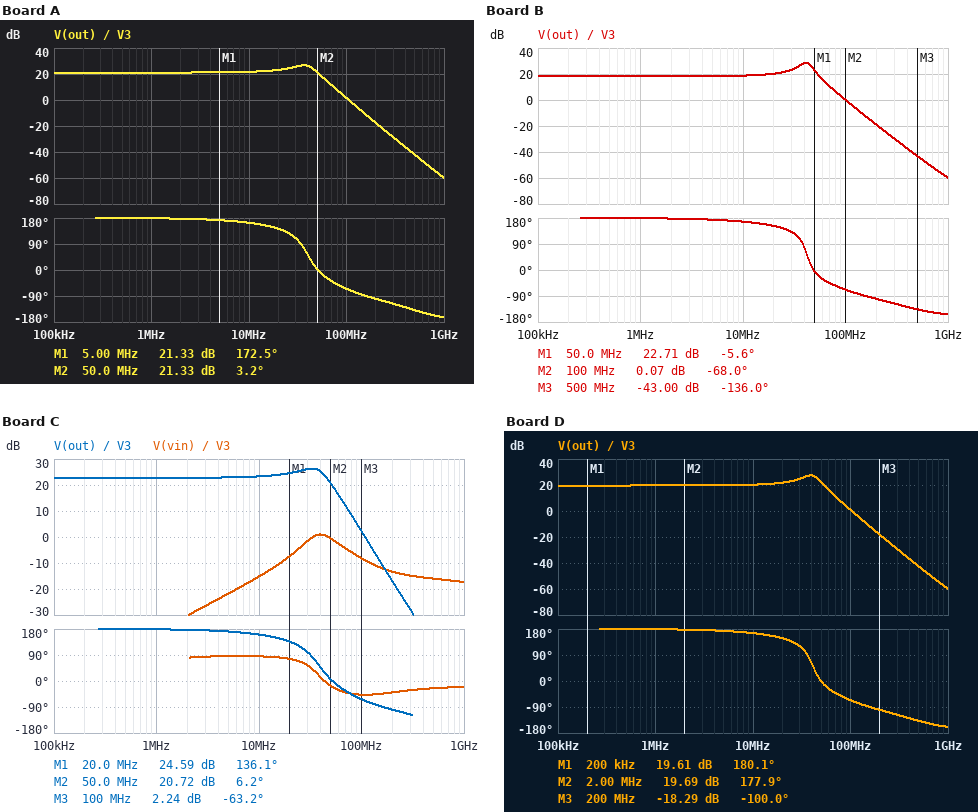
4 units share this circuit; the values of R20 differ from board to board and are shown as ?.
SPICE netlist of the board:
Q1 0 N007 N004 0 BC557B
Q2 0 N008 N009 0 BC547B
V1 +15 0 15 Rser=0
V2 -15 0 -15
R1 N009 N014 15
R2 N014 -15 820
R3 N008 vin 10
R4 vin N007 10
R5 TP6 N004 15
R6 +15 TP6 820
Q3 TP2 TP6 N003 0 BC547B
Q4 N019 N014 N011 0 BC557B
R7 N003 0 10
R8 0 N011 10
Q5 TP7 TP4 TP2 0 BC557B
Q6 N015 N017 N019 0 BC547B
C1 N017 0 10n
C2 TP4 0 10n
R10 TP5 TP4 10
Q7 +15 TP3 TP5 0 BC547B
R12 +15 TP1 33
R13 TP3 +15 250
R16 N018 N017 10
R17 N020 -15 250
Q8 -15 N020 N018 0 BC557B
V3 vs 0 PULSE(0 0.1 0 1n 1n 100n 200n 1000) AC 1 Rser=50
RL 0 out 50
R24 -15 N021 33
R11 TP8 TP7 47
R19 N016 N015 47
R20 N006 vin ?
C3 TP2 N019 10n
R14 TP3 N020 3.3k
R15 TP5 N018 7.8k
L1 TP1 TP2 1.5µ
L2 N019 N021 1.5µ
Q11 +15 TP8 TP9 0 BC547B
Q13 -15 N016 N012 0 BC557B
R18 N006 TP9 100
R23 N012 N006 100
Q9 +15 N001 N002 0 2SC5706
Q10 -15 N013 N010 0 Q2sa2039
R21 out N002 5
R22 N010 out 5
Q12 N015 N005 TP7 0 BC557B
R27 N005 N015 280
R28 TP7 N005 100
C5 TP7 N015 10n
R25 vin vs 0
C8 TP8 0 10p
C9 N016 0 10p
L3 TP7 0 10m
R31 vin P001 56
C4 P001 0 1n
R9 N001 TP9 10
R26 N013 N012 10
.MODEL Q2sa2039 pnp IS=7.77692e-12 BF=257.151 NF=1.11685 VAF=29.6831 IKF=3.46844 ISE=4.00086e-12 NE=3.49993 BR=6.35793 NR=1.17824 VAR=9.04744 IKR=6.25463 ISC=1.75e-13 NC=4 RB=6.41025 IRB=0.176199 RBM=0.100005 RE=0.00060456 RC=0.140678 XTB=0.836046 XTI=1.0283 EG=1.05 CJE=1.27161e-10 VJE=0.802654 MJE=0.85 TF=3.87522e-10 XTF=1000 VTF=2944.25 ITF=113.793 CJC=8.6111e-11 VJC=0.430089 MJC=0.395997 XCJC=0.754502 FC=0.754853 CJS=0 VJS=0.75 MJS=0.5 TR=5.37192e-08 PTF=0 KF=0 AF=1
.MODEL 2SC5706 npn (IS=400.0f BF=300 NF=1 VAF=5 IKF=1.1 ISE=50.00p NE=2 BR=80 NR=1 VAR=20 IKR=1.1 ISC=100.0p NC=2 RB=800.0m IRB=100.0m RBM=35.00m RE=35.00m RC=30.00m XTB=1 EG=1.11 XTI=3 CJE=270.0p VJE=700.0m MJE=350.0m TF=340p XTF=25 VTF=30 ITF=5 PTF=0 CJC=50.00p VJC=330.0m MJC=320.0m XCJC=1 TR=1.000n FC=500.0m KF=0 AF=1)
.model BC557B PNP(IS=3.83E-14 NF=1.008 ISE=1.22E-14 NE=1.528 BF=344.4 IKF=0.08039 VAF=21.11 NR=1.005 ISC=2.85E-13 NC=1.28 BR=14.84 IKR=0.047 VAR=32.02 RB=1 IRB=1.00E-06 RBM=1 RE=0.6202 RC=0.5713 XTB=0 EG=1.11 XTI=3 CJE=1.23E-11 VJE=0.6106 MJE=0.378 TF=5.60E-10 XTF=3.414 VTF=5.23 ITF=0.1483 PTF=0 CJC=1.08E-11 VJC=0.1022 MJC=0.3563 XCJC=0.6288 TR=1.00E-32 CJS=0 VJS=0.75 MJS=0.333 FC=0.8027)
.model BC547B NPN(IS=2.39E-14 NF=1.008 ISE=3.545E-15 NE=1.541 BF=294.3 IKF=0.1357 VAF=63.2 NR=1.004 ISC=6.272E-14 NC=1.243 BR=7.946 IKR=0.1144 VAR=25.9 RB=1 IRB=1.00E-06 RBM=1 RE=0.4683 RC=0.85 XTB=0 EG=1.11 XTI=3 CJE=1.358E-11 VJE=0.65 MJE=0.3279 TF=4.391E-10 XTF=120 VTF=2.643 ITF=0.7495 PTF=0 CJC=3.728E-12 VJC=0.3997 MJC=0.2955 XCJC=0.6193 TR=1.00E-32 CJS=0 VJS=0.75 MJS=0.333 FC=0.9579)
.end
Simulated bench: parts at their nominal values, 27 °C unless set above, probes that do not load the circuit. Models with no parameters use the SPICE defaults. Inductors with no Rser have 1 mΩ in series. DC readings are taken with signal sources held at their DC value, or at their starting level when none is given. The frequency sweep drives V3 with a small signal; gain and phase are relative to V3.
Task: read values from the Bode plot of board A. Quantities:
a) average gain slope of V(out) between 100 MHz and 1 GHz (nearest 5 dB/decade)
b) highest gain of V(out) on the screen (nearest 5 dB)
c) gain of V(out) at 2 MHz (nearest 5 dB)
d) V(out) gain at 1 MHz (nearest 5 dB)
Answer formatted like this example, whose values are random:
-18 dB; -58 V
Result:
-60 dB/decade; 25 dB; 20 dB; 20 dB
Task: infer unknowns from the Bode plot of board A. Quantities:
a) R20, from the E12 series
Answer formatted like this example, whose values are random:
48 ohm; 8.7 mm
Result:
560 Ω
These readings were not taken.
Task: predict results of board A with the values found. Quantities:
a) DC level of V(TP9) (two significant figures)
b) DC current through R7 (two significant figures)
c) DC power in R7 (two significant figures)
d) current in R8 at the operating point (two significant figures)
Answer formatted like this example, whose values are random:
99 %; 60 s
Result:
-680 mV; 16 mA; 2.4 mW; 35 mA
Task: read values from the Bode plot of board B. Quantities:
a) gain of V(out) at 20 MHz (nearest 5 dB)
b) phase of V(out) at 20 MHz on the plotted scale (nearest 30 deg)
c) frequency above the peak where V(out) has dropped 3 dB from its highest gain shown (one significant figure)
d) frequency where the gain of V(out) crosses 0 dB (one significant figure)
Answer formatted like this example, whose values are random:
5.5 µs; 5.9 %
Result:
20 dB; 150 deg; 50 MHz; 100 MHz
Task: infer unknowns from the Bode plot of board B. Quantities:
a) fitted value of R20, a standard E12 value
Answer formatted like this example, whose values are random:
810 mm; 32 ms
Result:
390 Ω
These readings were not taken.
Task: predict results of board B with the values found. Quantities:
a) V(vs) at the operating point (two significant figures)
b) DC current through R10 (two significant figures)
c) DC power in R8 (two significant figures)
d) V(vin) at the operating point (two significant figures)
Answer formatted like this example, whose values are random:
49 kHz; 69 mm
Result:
-140 mV; 110 µA; 14 mW; -140 mV
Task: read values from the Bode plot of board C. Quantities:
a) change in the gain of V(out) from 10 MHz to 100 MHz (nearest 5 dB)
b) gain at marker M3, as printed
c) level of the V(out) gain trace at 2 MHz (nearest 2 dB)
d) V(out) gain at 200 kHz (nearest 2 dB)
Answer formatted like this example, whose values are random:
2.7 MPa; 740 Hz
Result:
-20 dB; 2.24 dB; 22 dB; 22 dB
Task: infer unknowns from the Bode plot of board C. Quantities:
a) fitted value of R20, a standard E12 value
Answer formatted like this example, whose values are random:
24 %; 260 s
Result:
680 Ω
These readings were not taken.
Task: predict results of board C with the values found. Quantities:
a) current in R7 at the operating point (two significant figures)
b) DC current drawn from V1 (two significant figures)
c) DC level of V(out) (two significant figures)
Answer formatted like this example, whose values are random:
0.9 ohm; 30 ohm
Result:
17 mA; 96 mA; -1.3 V
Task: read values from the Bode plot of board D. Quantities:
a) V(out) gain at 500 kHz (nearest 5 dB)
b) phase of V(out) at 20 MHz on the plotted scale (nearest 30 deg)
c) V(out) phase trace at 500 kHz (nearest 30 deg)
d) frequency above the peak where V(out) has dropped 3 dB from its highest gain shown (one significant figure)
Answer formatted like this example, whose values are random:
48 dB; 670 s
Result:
20 dB; 150 deg; 180 deg; 50 MHz
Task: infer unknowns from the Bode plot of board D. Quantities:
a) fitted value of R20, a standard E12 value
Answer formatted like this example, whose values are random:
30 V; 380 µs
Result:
470 Ω
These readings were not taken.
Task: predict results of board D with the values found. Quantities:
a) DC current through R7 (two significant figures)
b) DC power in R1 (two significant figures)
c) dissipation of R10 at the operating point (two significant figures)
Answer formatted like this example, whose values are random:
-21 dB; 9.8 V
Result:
14 mA; 4.3 mW; 120 nW
